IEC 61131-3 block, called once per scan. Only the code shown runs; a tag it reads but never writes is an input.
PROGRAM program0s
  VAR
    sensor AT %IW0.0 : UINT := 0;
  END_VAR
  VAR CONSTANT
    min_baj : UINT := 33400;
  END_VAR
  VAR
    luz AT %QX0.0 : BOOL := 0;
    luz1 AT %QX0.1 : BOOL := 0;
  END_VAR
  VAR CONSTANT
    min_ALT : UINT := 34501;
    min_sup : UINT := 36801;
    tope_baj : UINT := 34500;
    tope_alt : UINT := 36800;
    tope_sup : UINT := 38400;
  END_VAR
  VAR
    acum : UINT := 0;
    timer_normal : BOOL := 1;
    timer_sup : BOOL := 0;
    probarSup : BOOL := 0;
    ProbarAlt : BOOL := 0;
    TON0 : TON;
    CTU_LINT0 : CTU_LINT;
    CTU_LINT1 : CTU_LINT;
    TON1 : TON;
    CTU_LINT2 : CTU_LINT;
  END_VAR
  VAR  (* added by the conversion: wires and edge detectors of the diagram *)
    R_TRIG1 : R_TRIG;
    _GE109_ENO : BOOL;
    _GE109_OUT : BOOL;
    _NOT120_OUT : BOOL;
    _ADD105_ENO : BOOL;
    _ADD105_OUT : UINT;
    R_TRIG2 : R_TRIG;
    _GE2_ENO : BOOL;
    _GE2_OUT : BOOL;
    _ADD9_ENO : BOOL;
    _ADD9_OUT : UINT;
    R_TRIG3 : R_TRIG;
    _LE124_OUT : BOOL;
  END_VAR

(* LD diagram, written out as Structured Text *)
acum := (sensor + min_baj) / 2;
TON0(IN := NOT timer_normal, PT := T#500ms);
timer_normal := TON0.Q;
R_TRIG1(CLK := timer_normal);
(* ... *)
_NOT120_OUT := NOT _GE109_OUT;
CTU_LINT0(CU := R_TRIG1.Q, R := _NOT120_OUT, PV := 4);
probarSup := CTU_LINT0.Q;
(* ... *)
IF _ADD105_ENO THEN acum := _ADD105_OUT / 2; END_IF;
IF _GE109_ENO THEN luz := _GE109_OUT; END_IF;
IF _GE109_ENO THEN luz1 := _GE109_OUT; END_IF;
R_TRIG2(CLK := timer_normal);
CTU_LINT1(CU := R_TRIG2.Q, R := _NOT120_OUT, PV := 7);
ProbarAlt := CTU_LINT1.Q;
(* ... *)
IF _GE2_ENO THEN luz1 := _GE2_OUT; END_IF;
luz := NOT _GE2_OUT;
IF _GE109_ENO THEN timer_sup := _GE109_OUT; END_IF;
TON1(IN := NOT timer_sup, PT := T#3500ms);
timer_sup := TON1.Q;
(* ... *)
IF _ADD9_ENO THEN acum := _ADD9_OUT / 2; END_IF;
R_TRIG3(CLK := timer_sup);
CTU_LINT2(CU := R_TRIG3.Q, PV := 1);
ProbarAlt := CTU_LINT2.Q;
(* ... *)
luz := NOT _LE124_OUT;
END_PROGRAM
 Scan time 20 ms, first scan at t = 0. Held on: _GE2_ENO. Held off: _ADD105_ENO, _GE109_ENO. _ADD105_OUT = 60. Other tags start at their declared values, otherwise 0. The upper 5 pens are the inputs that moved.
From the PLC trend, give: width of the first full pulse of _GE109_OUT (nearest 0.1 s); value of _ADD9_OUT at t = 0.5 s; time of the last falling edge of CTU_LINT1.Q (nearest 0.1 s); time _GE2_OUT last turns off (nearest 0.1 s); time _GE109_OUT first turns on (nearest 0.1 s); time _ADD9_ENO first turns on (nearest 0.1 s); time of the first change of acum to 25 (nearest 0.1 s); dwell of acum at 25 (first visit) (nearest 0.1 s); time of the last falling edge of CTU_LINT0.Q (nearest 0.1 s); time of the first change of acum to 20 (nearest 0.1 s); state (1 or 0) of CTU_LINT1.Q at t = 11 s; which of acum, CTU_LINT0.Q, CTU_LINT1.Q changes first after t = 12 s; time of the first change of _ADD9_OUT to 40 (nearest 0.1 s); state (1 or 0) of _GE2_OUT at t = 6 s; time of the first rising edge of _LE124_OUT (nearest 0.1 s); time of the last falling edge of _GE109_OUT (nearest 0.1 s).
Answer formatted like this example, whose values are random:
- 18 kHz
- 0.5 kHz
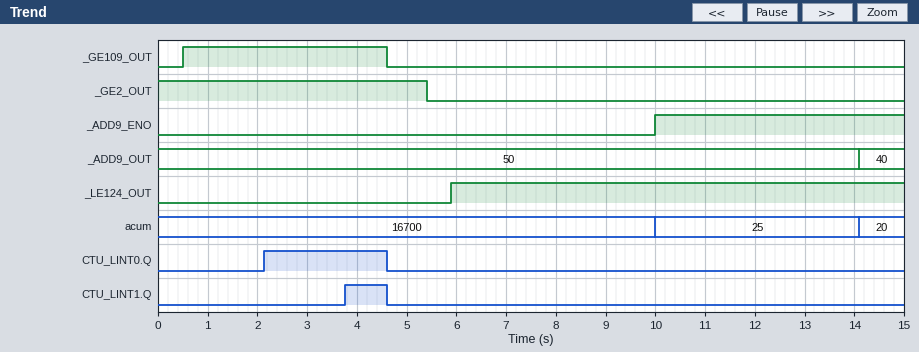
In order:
- 4.1 s
- 50
- 4.6 s
- 5.4 s
- 0.5 s
- 10.0 s
- 10.0 s
- 4.1 s
- 4.6 s
- 14.1 s
- 0
- acum
- 14.1 s
- 0
- 5.9 s
- 4.6 s
